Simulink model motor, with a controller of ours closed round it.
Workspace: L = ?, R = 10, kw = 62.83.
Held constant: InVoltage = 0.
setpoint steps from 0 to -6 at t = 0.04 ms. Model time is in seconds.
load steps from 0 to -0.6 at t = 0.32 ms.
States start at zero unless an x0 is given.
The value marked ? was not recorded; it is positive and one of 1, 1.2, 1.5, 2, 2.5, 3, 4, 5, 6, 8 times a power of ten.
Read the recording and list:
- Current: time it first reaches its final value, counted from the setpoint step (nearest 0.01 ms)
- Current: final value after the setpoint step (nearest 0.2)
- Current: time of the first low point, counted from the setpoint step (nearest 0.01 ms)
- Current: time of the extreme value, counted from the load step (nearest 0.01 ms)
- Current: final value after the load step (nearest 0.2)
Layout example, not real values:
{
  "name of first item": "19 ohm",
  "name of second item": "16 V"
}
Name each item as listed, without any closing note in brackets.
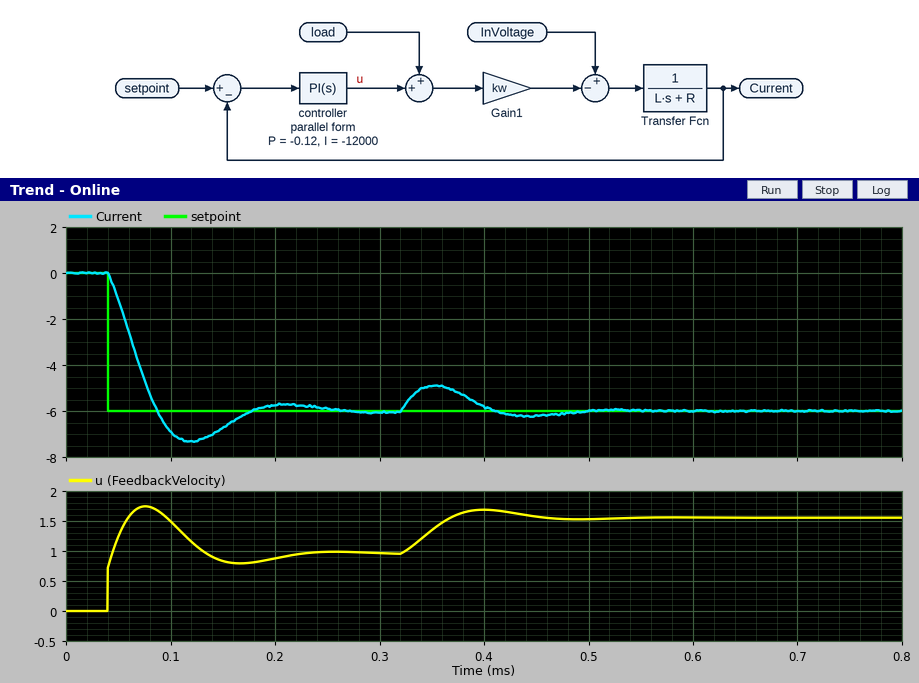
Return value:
{
  "Current: time it first reaches its final value, counted from the setpoint step": "0.05 ms",
  "Current: final value after the setpoint step": "-6.0",
  "Current: time of the first low point, counted from the setpoint step": "0.08 ms",
  "Current: time of the extreme value, counted from the load step": "0.03 ms",
  "Current: final value after the load step": "-6.0"
}
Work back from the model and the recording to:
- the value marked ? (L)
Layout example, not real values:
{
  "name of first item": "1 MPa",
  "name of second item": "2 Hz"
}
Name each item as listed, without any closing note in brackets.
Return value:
{
  "the value marked ?": "0.0005"
}
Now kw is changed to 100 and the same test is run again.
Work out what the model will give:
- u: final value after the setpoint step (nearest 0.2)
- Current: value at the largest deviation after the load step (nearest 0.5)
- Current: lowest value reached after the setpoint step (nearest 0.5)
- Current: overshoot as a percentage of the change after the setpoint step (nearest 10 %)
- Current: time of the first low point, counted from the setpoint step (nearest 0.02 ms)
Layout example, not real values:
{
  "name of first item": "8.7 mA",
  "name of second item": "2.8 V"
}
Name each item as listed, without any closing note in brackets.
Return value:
{
  "u: final value after the setpoint step": "0.6",
  "Current: value at the largest deviation after the load step": "-4.5",
  "Current: lowest value reached after the setpoint step": "-7.5",
  "Current: overshoot as a percentage of the change after the setpoint step": "20 %",
  "Current: time of the first low point, counted from the setpoint step": "0.06 ms"
}
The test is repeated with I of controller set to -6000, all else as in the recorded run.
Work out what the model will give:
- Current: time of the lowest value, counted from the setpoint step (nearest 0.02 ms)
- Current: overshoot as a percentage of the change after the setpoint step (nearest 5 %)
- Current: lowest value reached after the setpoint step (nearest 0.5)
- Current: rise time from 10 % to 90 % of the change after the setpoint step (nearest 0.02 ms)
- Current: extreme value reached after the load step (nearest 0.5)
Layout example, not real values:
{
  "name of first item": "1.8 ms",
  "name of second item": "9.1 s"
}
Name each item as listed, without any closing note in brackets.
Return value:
{
  "Current: time of the lowest value, counted from the setpoint step": "0.12 ms",
  "Current: overshoot as a percentage of the change after the setpoint step": "10 %",
  "Current: lowest value reached after the setpoint step": "-6.5",
  "Current: rise time from 10 % to 90 % of the change after the setpoint step": "0.06 ms",
  "Current: extreme value reached after the load step": "-4.5"
}
